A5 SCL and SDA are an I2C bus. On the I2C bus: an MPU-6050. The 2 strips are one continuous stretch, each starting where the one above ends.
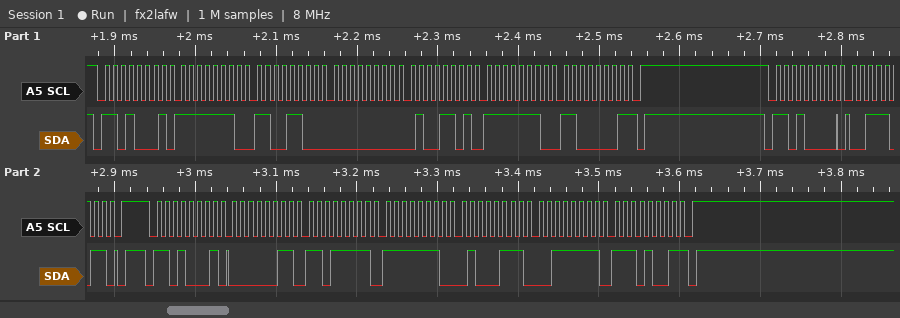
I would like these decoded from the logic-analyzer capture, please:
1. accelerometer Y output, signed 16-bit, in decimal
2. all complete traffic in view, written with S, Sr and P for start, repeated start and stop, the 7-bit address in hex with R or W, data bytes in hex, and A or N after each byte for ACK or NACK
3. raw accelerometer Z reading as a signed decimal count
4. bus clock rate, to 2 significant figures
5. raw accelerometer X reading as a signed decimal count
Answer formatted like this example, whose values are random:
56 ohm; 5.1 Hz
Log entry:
-441; S 68R A FE A CC A 00 A 4D A FE A C1 N P S 68W A 3B A P S 68R A 03 A DF A FE A 47 A 3F A E9 N P; 16361; 100 kHz; 991
